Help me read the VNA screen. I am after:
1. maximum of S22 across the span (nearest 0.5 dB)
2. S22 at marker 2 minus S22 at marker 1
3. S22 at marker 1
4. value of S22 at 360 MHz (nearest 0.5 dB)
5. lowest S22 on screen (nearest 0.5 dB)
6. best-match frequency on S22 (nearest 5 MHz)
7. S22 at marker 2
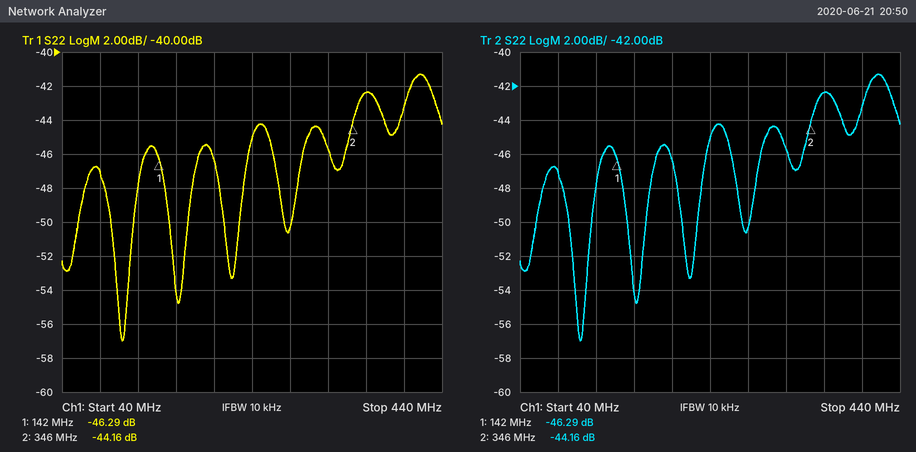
-41.5 dB
2.13 dB
-46.29 dB
-42.5 dB
-57.0 dB
105 MHz
-44.16 dB
